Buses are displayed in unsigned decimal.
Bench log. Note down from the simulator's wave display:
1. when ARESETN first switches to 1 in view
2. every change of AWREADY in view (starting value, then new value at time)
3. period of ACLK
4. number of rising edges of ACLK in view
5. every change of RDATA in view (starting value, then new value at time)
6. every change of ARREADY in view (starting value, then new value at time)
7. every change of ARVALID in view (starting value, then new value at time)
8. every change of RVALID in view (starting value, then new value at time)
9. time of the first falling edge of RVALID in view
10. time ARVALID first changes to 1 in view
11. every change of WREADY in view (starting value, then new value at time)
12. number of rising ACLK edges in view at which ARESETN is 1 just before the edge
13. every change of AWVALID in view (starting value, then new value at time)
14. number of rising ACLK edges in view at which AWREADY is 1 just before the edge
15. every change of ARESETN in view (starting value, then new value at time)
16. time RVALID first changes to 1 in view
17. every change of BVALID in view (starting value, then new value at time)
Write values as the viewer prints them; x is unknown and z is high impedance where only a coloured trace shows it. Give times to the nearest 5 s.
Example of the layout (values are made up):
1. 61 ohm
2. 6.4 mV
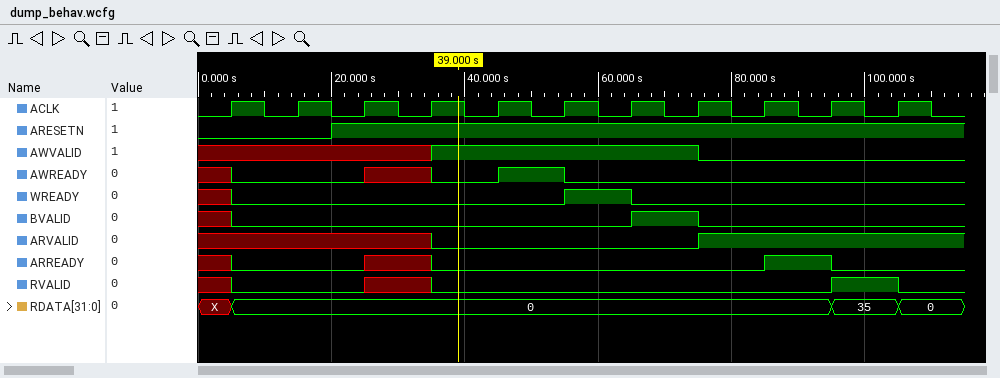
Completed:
1. 20 s
2. x, 0 at 5 s, x at 25 s, 0 at 35 s, 1 at 45 s, 0 at 55 s
3. 10 s
4. 11
5. X, 0 at 5 s, 35 at 95 s, 0 at 105 s
6. x, 0 at 5 s, x at 25 s, 0 at 35 s, 1 at 85 s, 0 at 95 s
7. x, 0 at 35 s, 1 at 75 s
8. x, 0 at 5 s, x at 25 s, 0 at 35 s, 1 at 95 s, 0 at 105 s
9. 105 s
10. 75 s
11. x, 0 at 5 s, 1 at 55 s, 0 at 65 s
12. 9
13. x, 1 at 35 s, 0 at 75 s
14. 1
15. 0, 1 at 20 s
16. 95 s
17. x, 0 at 5 s, 1 at 65 s, 0 at 75 s
